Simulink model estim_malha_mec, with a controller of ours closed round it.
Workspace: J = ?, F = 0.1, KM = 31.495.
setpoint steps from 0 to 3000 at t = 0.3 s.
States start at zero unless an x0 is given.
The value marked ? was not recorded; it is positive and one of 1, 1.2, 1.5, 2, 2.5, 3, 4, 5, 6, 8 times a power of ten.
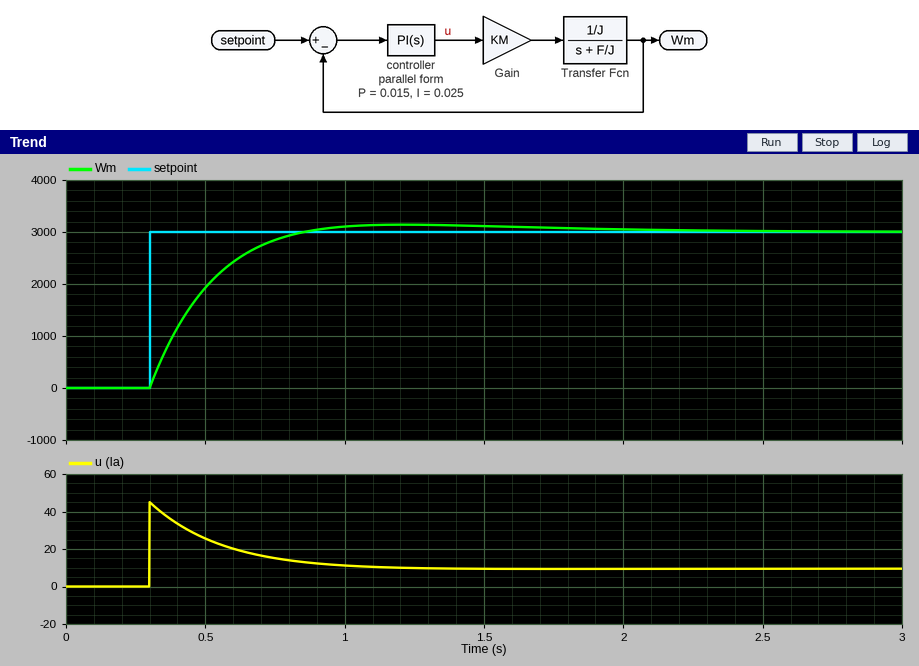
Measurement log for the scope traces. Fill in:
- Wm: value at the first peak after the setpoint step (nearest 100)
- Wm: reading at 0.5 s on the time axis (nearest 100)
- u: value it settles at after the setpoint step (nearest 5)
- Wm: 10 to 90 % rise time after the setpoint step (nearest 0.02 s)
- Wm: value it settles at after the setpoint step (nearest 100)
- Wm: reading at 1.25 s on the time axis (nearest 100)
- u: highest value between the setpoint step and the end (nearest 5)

3100
1900
10
0.36 s
3000
3100
45
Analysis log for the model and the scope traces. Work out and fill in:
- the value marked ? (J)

0.1
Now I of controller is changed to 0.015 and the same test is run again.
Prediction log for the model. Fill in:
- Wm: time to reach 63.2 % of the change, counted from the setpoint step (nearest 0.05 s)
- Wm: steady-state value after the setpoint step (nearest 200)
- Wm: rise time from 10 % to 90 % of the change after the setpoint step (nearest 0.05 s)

0.20 s
3000
0.45 s
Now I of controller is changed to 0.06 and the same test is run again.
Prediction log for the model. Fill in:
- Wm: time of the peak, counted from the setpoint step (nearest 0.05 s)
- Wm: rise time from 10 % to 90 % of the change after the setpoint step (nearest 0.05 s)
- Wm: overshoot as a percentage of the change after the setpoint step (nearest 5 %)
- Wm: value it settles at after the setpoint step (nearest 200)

0.60 s
0.25 s
15 %
3000
